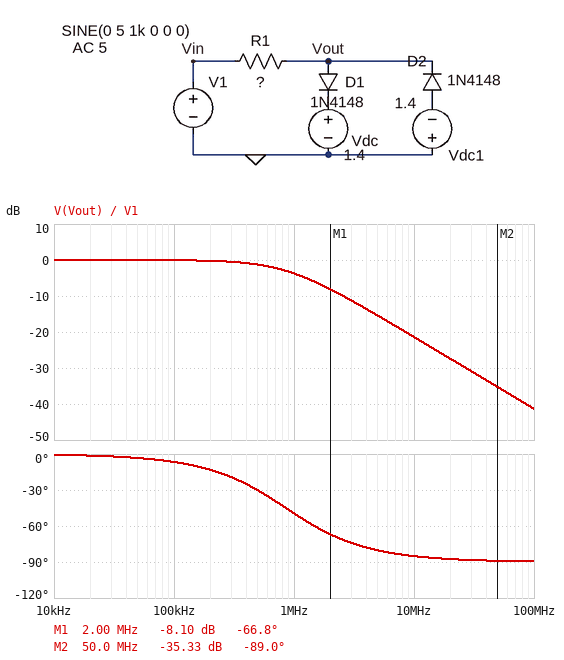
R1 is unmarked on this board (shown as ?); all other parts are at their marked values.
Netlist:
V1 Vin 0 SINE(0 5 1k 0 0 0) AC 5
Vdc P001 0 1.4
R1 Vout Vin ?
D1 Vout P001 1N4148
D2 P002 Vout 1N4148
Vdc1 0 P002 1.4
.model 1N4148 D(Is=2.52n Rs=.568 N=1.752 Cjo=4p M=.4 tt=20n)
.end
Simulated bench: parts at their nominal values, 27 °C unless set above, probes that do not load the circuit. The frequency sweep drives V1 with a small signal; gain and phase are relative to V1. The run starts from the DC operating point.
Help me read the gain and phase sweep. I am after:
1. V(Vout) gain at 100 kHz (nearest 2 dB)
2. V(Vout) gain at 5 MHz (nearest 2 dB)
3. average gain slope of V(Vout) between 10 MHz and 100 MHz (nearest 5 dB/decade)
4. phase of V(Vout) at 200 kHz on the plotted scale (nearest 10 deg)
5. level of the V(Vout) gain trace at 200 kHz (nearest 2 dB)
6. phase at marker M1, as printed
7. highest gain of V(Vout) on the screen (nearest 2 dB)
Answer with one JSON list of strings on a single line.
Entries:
["0 dB", "-16 dB", "-20 dB/decade", "-10 deg", "0 dB", "-66.8 deg", "0 dB"]
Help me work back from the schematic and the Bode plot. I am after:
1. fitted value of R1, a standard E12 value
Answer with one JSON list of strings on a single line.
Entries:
["33 kΩ"]
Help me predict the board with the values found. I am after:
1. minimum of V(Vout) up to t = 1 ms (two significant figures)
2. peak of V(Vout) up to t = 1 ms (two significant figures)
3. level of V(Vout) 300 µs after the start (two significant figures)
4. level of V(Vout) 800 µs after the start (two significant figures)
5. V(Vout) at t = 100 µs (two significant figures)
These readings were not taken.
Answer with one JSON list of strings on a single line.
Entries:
["-1.9 V", "1.9 V", "1.9 V", "-1.9 V", "1.8 V"]
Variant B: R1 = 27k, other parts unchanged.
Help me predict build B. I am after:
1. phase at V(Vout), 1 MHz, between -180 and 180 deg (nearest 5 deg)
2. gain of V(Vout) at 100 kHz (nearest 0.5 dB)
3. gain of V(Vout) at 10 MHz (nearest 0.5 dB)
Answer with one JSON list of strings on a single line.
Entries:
["-45 deg", "0 dB", "-19.5 dB"]
